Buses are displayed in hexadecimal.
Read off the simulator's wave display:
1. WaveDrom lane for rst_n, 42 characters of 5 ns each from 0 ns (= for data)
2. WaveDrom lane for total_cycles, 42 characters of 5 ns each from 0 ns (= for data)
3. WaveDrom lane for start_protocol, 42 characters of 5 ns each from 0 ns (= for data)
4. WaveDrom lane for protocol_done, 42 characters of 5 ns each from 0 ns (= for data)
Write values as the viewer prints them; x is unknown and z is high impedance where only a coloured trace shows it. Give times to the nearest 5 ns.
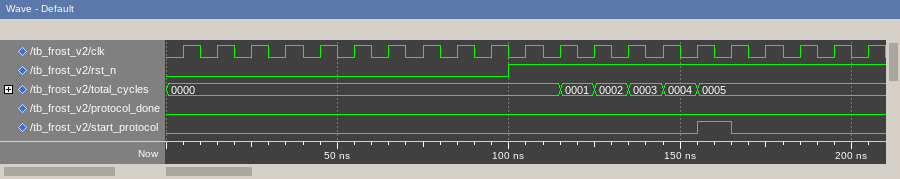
{name: 'rst_n', wave: '0...................1.....................'}
{name: 'total_cycles', wave: '=......................=.=.=.=.=..........', data: '0000 0001 0002 0003 0004 0005'}
{name: 'start_protocol', wave: '0..............................1.0........'}
{name: 'protocol_done', wave: '0.........................................'}
